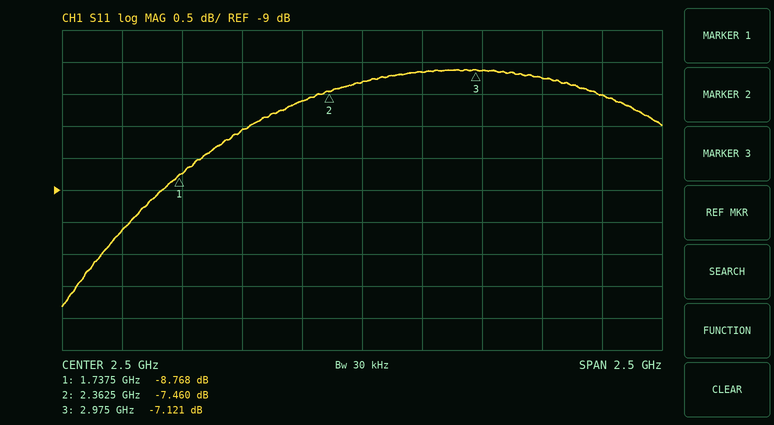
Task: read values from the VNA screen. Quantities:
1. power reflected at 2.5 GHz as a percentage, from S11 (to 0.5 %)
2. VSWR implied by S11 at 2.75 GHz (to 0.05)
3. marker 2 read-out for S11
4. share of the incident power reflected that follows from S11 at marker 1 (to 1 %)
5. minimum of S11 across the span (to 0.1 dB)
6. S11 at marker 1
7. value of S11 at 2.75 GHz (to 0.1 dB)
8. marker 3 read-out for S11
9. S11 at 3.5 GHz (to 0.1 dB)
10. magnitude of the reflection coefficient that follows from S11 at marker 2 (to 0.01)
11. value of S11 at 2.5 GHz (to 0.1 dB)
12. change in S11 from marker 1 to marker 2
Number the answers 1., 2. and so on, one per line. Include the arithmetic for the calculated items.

1. 10^(-7.3/10) ≈ 18.6 %, so 18.5 % to the nearest 0.5 %
2. |Γ| = 10^(-7.2/20) = 0.4365; VSWR = (1 + 0.4365)/(1 − 0.4365) ≈ 2.55
3. -7.460 dB
4. 10^(-8.768/10) ≈ 13 %
5. -10.8 dB
6. -8.768 dB
7. -7.2 dB
8. -7.121 dB
9. -7.5 dB
10. 10^(-7.46/20) ≈ 0.42
11. -7.3 dB
12. -7.46 − (-8.768) = 1.308 dB
